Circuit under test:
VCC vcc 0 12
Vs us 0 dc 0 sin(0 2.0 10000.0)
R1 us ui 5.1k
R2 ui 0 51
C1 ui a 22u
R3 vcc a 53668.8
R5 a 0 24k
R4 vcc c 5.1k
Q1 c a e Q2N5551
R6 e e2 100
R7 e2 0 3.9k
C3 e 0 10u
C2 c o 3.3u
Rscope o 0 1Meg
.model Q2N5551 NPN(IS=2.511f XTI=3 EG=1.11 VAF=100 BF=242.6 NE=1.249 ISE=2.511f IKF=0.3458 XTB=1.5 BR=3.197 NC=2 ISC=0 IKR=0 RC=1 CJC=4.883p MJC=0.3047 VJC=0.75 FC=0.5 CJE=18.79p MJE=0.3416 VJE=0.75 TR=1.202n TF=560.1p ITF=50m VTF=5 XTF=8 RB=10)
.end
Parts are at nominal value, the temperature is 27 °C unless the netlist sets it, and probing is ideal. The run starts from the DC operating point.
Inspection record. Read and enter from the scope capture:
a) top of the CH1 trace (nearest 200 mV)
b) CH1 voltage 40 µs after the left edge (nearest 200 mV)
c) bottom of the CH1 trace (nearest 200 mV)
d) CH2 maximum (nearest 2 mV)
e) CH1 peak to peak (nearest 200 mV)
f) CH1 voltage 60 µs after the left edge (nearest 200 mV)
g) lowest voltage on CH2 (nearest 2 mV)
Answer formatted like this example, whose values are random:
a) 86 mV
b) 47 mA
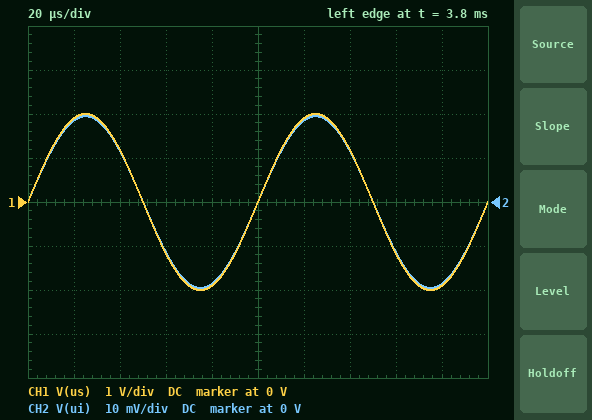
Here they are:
a) 2.0 V
b) 1.2 V
c) -2.0 V
d) 20 mV
e) 4.0 V
f) -1.2 V
g) -20 mV
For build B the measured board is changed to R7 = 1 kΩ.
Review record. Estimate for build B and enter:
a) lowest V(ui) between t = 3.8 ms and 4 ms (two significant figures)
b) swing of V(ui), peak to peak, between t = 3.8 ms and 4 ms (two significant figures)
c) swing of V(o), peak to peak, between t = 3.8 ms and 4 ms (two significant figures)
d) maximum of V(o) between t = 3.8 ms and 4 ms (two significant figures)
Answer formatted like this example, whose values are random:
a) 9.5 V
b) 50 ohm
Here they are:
a) -18 mV
b) 25 mV
c) 3.0 V
d) 2.9 V
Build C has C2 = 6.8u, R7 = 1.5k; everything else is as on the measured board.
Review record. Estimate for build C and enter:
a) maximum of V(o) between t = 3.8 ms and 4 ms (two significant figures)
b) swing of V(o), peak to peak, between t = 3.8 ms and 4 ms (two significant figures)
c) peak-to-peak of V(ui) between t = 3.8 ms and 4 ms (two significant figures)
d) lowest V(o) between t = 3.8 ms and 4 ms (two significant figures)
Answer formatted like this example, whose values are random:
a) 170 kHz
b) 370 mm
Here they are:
a) 3.3 V
b) 3.8 V
c) 28 mV
d) -500 mV
